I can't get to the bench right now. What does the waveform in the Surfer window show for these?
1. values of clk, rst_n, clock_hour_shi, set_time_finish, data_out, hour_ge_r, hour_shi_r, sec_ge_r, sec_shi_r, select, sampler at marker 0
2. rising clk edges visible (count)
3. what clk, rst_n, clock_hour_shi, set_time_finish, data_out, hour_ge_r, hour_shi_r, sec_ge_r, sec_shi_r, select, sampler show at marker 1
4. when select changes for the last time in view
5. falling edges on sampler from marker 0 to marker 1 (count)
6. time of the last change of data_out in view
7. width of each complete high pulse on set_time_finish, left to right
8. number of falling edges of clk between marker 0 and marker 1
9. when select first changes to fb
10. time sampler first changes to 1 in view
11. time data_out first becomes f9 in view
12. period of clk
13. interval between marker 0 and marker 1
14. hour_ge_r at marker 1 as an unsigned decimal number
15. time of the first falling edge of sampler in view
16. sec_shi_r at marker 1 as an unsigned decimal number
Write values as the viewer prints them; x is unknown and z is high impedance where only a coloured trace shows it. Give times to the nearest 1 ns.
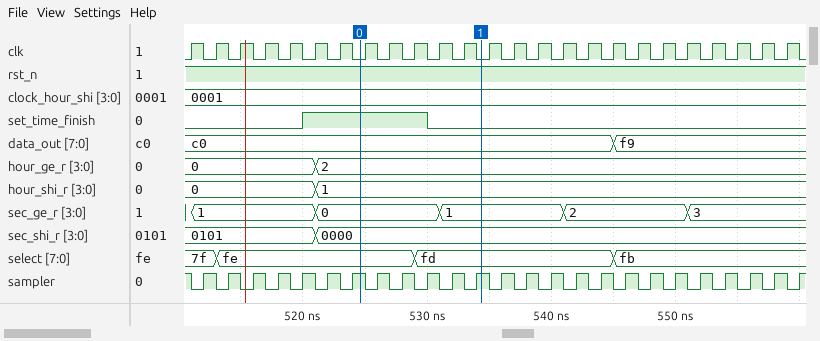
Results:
clk=0, rst_n=1, clock_hour_shi=0001, set_time_finish=1, data_out=c0, hour_ge_r=2, hour_shi_r=1, sec_ge_r=0, sec_shi_r=0000, select=fe, sampler=1
25
clk=0, rst_n=1, clock_hour_shi=0001, set_time_finish=0, data_out=c0, hour_ge_r=2, hour_shi_r=1, sec_ge_r=1, sec_shi_r=0000, select=fd, sampler=1
545 ns
5
545 ns
10 ns
5
545 ns
512 ns
545 ns
2 ns
10 ns
2
511 ns
0
